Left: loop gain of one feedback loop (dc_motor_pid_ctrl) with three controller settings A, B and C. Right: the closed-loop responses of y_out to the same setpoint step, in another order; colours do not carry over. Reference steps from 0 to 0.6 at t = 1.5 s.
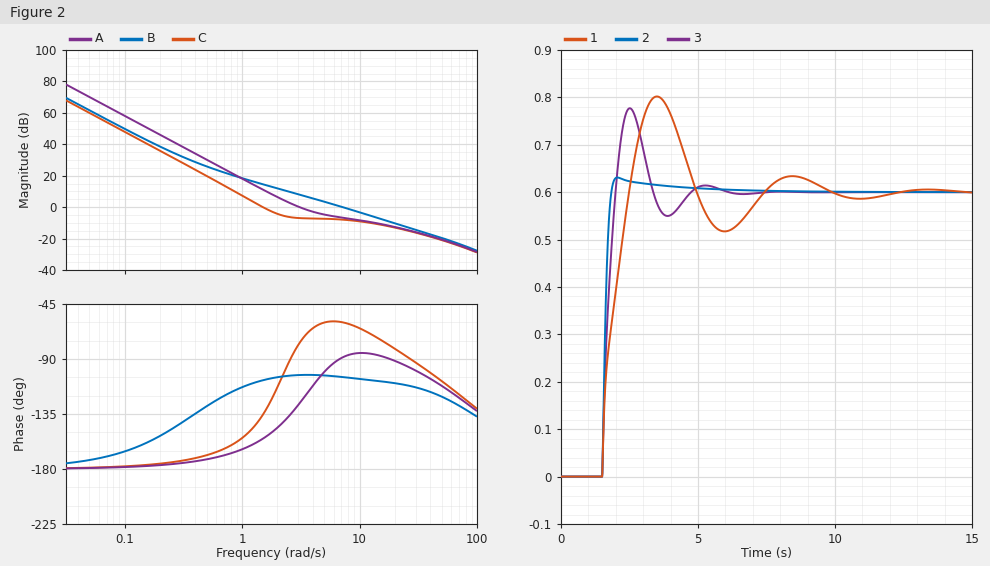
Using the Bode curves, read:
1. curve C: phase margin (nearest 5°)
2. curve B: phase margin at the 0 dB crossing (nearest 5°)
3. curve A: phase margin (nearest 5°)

45°
75°
55°
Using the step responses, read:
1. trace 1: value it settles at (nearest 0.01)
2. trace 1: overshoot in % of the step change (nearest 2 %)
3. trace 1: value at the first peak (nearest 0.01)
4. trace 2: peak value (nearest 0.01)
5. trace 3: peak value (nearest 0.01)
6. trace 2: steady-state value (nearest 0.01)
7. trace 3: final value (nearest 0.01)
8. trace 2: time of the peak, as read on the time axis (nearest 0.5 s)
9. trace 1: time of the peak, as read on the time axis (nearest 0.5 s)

0.60
34 %
0.80
0.63
0.78
0.60
0.60
2.0 s
3.5 s
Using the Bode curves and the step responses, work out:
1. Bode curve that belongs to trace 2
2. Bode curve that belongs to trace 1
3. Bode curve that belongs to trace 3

B
C
A
